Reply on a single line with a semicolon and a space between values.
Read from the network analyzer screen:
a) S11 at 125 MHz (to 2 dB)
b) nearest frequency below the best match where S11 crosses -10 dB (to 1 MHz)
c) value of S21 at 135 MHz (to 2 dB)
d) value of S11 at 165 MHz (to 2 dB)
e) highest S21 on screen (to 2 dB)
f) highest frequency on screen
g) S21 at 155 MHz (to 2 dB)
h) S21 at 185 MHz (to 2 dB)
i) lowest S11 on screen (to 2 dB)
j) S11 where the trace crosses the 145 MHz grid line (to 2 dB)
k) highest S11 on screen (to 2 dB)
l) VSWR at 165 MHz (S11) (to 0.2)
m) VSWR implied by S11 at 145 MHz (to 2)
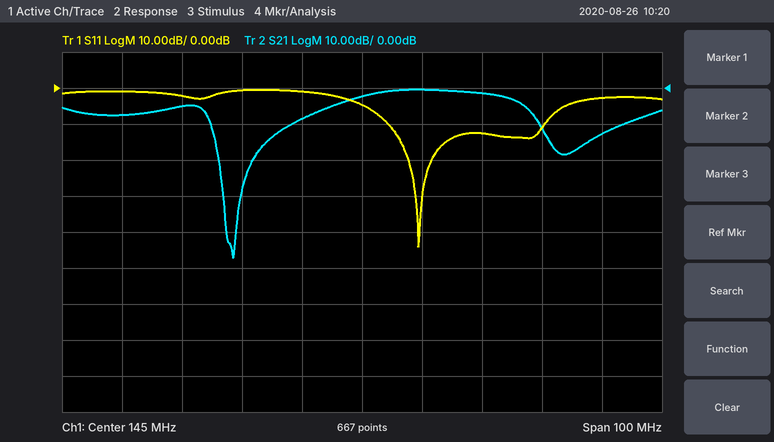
0 dB; 149 MHz; -8 dB; -12 dB; 0 dB; 195 MHz; 0 dB; -12 dB; -44 dB; -4 dB; 0 dB; 1.6; 4
